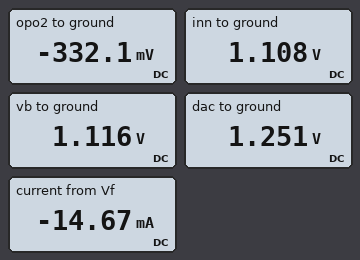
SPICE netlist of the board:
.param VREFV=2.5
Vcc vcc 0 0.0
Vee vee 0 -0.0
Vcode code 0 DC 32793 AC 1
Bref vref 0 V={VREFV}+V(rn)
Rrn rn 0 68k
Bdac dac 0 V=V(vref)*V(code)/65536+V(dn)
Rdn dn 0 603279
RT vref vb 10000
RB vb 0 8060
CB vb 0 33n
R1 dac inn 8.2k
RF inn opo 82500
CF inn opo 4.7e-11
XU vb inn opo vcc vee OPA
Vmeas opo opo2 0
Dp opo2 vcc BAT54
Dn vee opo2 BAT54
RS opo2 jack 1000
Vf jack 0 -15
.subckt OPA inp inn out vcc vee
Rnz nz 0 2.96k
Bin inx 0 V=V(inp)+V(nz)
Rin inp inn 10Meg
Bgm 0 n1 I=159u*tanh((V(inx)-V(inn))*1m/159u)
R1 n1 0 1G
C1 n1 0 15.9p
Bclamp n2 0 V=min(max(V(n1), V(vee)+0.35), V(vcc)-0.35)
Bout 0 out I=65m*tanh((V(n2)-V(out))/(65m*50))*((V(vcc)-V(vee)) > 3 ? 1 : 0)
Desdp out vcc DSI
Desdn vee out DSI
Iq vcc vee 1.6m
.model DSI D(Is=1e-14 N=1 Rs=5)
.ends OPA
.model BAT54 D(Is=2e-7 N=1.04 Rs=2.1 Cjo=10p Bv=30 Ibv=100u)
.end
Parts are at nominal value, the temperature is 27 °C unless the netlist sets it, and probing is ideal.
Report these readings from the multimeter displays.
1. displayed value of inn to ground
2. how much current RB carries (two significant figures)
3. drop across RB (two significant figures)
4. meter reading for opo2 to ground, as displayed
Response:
1.108 V
140 µA
1.1 V
-332.1 mV
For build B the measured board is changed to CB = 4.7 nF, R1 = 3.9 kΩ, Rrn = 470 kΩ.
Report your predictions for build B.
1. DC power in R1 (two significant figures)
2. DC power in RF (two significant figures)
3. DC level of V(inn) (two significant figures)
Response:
1.3 µW
28 µW
1.2 V
